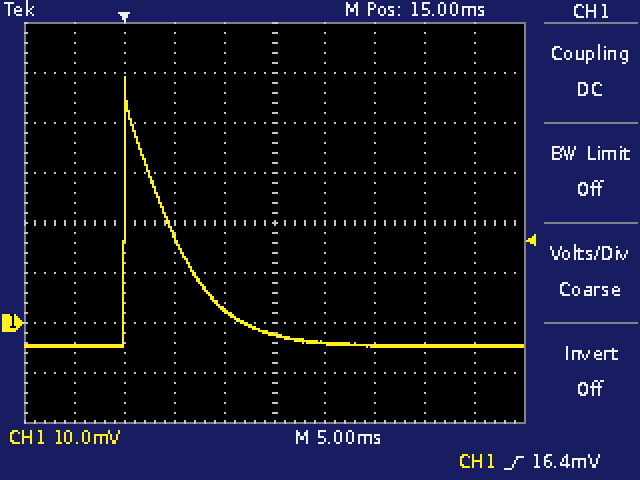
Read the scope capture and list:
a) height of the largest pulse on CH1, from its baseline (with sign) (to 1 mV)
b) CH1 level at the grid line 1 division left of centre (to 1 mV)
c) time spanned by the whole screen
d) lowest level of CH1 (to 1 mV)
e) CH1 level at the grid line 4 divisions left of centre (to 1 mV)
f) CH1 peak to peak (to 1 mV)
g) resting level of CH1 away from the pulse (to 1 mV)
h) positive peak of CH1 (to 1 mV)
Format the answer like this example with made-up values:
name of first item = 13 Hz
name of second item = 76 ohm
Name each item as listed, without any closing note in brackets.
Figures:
height of the largest pulse on CH1, from its baseline (with sign) = +54 mV
CH1 level at the grid line 1 division left of centre = 3 mV
time spanned by the whole screen = 50 ms
lowest level of CH1 = -5 mV
CH1 level at the grid line 4 divisions left of centre = -5 mV
CH1 peak to peak = 54 mV
resting level of CH1 away from the pulse = -5 mV
positive peak of CH1 = 49 mV
